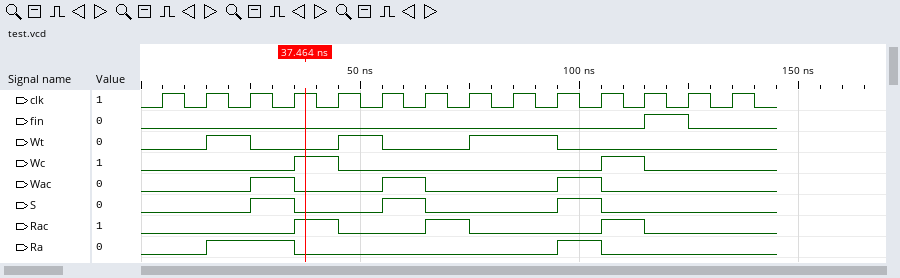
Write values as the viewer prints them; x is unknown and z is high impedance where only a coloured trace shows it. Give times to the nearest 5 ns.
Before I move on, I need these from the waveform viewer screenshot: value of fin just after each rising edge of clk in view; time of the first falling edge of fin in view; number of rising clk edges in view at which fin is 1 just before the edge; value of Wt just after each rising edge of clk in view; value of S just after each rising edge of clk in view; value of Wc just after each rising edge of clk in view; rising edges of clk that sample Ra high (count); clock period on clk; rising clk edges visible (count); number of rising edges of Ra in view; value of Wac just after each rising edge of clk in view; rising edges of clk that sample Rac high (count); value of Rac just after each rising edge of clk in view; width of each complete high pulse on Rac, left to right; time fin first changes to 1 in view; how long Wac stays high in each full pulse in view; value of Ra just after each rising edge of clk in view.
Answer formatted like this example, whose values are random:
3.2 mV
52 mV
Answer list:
0 0 0 0 0 0 0 0 0 0 0 1 0 0
125 ns
1
0 1 0 0 1 0 0 1 1 0 0 0 0 0
0 0 1 0 0 1 0 0 0 1 0 0 0 0
0 0 0 1 0 0 0 0 0 0 1 0 0 0
3
10 ns
14
2
0 0 1 0 0 1 0 0 0 1 0 0 0 0
3
0 0 0 1 0 0 1 0 0 0 1 0 0 0
10 ns, 10 ns, 10 ns
115 ns
10 ns, 10 ns, 10 ns
0 1 1 0 0 0 0 0 0 1 0 0 0 0
